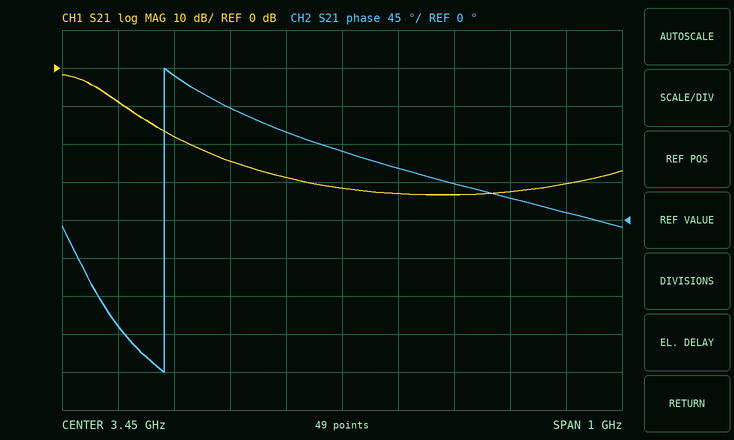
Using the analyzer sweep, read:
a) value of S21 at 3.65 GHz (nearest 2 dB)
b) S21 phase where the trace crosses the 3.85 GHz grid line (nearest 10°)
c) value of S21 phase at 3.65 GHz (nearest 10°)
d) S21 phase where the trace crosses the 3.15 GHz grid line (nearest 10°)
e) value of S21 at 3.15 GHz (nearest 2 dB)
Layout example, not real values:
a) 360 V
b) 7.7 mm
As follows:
a) -34 dB
b) 10°
c) 40°
d) 170°
e) -18 dB
